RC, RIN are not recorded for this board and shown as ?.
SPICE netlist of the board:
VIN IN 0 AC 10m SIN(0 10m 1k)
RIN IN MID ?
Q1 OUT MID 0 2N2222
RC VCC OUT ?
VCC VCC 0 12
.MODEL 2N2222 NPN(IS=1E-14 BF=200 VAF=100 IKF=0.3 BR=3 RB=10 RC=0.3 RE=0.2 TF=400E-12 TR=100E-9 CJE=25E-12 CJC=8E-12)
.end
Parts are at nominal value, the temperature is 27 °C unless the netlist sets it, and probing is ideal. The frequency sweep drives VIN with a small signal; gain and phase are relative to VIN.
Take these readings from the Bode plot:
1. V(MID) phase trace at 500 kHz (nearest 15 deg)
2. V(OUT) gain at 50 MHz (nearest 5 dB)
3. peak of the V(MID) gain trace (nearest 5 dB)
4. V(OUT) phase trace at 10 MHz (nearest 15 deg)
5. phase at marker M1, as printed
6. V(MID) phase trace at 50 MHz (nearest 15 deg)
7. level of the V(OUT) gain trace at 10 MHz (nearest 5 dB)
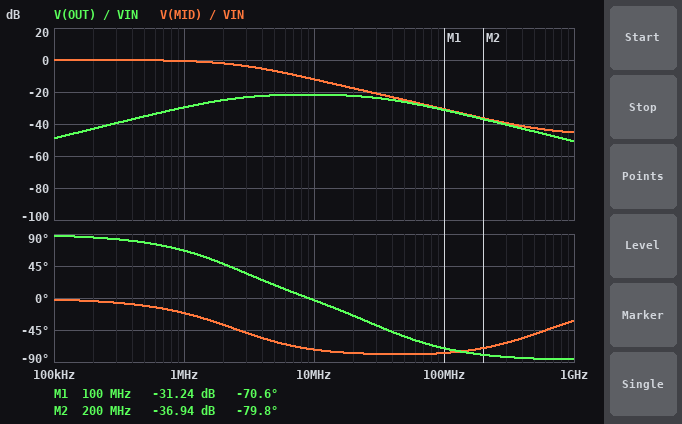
-15 deg
-25 dB
0 dB
0 deg
-70.6 deg
-75 deg
-20 dB
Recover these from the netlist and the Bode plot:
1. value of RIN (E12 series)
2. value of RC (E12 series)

2.2 kΩ
1.8 kΩ
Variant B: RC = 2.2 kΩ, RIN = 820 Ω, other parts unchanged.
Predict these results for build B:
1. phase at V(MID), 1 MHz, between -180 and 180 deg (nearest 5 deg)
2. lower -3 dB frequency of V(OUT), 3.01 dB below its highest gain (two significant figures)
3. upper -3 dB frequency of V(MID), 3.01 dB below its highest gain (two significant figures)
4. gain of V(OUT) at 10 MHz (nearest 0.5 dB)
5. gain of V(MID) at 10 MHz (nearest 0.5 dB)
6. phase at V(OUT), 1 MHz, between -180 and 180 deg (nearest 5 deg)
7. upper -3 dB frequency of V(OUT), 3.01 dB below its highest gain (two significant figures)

-10 deg
4.6 MHz
6.7 MHz
-13.0 dB
-5.0 dB
80 deg
38 MHz
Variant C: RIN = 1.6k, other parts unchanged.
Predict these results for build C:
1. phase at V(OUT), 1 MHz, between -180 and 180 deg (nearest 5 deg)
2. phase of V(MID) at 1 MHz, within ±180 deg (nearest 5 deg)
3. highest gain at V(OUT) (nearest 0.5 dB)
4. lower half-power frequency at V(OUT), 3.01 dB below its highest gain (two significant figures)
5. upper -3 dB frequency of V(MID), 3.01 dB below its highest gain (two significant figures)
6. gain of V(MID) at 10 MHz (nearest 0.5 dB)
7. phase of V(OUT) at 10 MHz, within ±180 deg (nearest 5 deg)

70 deg
-15 deg
-19.0 dB
2.9 MHz
3.5 MHz
-9.5 dB
0 deg
